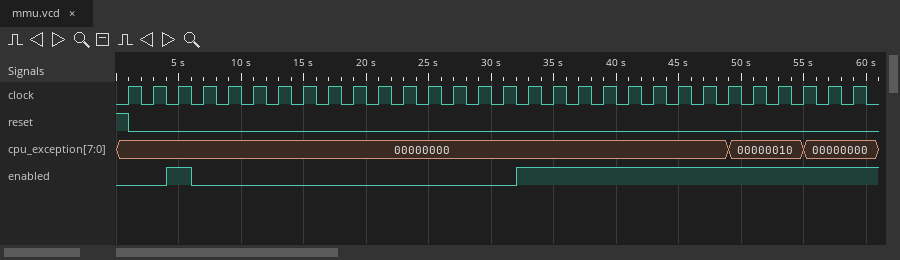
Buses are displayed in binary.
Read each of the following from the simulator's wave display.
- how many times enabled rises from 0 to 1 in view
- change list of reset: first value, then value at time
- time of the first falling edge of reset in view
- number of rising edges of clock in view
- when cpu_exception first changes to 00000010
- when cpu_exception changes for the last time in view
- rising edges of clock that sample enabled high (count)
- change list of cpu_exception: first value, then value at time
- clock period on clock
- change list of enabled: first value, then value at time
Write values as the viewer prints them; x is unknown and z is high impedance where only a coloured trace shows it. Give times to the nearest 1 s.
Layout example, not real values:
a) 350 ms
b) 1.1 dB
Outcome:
a) 2
b) 1, 0 at 1 s
c) 1 s
d) 30
e) 49 s
f) 55 s
g) 15
h) 00000000, 00000010 at 49 s, 00000000 at 55 s
i) 2 s
j) 0, 1 at 4 s, 0 at 6 s, 1 at 32 s
